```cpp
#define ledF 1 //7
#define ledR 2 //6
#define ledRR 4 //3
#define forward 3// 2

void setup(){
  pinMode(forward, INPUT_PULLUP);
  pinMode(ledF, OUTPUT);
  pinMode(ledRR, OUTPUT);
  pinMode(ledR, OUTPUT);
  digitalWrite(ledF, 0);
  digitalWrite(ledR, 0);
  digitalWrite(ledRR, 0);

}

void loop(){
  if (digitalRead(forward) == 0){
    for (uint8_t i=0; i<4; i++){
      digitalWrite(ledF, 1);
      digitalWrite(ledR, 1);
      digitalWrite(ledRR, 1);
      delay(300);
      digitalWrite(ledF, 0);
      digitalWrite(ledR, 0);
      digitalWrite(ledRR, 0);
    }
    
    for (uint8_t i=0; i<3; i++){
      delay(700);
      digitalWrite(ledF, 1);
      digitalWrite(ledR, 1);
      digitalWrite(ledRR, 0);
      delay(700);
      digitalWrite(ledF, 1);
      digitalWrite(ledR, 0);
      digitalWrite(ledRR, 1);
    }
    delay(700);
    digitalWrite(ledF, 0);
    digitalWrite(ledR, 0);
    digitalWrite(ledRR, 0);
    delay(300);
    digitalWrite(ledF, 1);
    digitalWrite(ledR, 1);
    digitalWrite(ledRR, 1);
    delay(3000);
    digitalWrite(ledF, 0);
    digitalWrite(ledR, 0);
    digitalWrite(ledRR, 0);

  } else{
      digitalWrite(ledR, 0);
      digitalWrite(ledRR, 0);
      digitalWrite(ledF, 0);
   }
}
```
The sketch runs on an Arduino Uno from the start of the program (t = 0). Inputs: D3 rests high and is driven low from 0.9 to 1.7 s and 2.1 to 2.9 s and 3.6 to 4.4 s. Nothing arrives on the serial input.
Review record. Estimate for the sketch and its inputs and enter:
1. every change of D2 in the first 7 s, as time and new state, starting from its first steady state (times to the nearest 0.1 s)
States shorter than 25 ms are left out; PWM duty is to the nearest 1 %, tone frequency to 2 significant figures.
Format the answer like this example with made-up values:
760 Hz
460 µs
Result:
0 s low; 0.9 s high; 2.1 s low; 2.8 s high; 3.5 s low; 4.2 s high; 4.9 s low; 5.6 s high; 6.3 s low
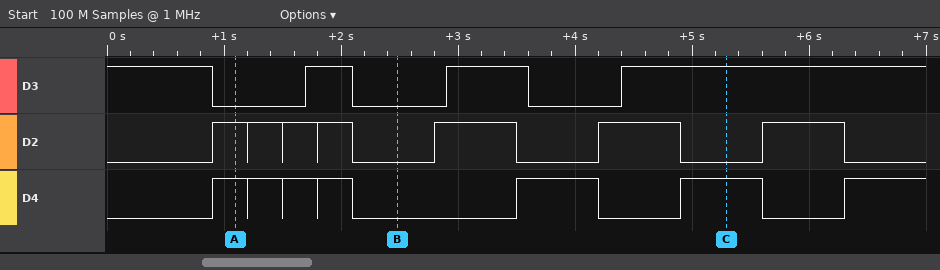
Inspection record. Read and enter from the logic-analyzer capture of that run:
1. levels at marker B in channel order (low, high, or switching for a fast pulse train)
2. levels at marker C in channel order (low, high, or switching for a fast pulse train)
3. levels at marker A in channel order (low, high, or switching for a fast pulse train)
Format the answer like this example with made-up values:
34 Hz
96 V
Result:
D3 low, D2 low, D4 low
D3 high, D2 low, D4 high
D3 low, D2 high, D4 high
